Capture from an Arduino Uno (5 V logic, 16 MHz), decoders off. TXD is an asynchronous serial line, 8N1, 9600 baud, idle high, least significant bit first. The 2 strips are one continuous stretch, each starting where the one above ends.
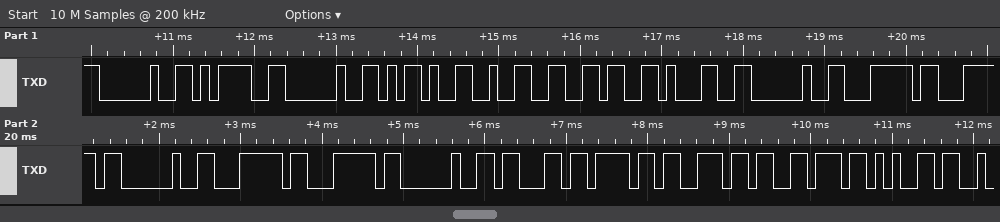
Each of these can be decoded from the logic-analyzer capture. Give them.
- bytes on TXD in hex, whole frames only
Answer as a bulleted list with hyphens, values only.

- 20 3D 20 2D 32 36 31 20 7C 7C 20 7C 7C 20 63 6F 6E 76 65
